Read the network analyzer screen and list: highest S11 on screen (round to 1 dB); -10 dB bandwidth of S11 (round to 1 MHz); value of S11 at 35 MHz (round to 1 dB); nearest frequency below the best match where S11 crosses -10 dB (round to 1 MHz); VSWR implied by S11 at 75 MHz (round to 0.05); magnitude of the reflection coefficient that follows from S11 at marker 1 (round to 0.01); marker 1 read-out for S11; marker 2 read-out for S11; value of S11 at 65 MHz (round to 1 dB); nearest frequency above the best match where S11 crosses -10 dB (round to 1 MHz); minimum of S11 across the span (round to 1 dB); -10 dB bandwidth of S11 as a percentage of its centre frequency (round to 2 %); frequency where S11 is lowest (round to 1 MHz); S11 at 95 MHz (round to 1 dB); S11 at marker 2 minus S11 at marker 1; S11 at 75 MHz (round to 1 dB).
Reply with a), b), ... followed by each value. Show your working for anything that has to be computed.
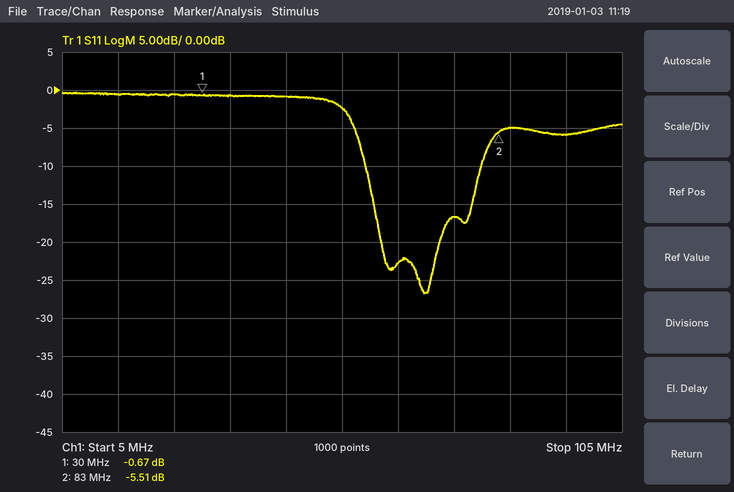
a) 0 dB
b) 80 MHz − 59 MHz = 21 MHz
c) -1 dB
d) 59 MHz
e) |Γ| = 10^(-17/20) = 0.1413; VSWR = (1 + 0.1413)/(1 − 0.1413) ≈ 1.33, so 1.35 to the nearest 0.05
f) 10^(-0.67/20) ≈ 0.93
g) -0.67 dB
h) -5.51 dB
i) -23 dB
j) 80 MHz
k) -27 dB
l) 21 MHz / 69.5 MHz ≈ 30 %
m) 70 MHz
n) -6 dB
o) -5.51 − (-0.67) = -4.84 dB
p) -17 dB
